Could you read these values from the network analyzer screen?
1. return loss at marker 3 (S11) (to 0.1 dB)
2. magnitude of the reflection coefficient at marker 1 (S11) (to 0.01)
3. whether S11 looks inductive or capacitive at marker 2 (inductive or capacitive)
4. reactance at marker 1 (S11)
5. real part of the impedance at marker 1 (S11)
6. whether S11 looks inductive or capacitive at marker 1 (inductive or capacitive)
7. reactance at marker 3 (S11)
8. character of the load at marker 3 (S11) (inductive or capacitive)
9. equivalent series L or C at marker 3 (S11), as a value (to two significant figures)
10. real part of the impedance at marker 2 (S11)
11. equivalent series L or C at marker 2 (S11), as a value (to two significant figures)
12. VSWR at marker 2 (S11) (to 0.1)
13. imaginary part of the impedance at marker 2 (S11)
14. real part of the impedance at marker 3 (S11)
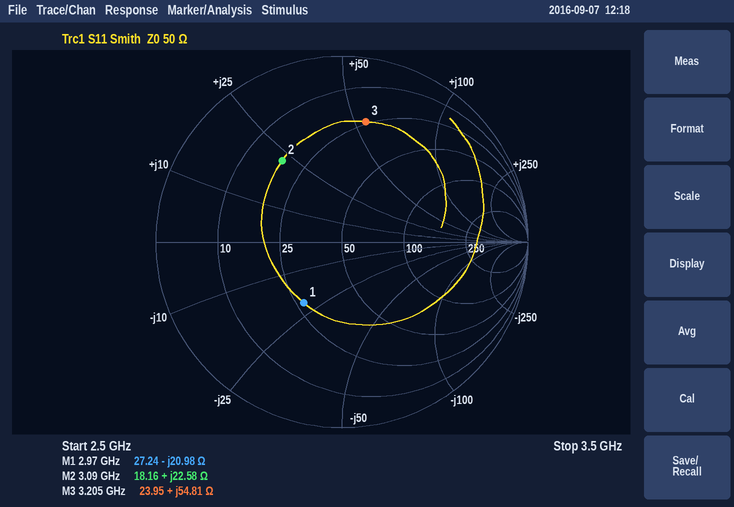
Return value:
3.6 dB
0.39
inductive
-20.98 Ω
27.24 Ω
capacitive
+54.81 Ω
inductive
2.7 nH
18.16 Ω
1.2 nH
3.4
+22.58 Ω
23.95 Ω
